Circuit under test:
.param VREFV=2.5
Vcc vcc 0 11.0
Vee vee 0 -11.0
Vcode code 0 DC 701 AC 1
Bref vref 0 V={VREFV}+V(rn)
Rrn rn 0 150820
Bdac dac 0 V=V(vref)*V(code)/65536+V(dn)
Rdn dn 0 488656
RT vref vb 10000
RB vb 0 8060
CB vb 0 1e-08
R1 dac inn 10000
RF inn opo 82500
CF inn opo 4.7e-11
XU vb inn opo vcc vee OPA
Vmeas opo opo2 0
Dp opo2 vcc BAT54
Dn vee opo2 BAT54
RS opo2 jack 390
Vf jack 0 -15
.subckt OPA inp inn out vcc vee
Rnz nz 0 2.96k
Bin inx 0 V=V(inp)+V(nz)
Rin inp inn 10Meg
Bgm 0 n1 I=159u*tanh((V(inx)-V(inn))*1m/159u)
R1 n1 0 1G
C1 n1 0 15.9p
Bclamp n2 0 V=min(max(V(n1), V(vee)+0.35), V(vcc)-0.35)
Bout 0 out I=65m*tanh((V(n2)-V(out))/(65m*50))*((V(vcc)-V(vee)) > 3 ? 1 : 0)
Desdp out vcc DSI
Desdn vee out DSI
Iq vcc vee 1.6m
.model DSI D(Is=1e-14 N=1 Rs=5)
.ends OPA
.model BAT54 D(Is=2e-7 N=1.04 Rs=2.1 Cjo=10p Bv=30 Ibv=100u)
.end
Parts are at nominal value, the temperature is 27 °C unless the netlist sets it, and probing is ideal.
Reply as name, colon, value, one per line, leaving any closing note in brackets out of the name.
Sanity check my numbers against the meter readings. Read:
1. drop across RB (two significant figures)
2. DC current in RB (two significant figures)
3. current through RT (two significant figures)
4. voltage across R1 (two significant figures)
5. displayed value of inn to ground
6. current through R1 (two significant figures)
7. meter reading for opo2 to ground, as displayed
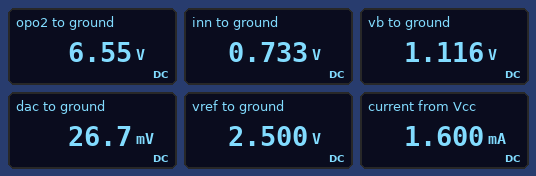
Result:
drop across RB: 1.1 V
DC current in RB: 140 µA
current through RT: 140 µA
voltage across R1: 710 mV
displayed value of inn to ground: 0.733 V
current through R1: 71 µA
meter reading for opo2 to ground, as displayed: 6.55 V
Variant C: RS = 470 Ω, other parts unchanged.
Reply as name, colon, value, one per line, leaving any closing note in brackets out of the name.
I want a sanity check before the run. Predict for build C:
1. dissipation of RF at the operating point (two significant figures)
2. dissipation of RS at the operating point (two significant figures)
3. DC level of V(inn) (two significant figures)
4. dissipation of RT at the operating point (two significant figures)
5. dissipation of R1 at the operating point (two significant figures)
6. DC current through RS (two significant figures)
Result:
dissipation of RF at the operating point: 550 µW
dissipation of RS at the operating point: 1.1 W
DC level of V(inn): 840 mV
dissipation of RT at the operating point: 190 µW
dissipation of R1 at the operating point: 66 µW
DC current through RS: 48 mA
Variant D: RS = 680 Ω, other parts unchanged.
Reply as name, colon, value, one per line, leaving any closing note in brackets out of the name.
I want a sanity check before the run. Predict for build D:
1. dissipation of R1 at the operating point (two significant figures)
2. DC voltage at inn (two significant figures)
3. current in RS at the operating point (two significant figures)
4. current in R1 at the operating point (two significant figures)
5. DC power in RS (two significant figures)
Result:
dissipation of R1 at the operating point: 88 µW
DC voltage at inn: 960 mV
current in RS at the operating point: 35 mA
current in R1 at the operating point: 94 µA
DC power in RS: 830 mW
